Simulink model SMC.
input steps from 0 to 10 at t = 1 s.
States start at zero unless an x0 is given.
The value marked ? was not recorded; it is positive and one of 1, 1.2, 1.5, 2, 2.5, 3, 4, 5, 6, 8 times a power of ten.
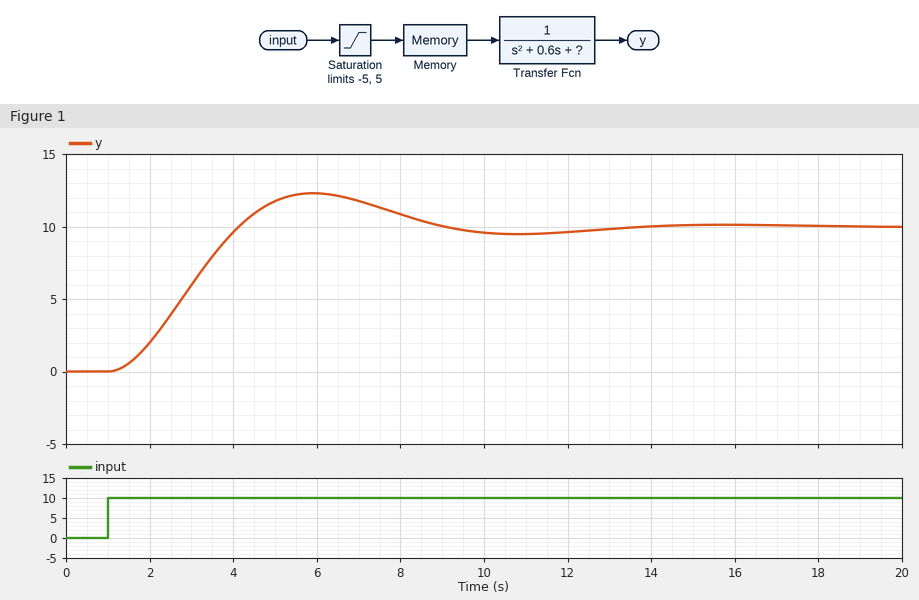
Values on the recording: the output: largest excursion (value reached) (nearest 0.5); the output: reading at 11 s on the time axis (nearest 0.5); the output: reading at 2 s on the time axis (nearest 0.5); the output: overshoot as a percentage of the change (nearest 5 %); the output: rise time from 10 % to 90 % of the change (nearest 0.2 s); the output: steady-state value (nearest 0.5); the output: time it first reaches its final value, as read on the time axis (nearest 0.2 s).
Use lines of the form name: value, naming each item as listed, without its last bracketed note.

the output: largest excursion (value reached): 12.5
the output: reading at 11 s on the time axis: 9.5
the output: reading at 2 s on the time axis: 2.0
the output: overshoot as a percentage of the change: 25 %
the output: rise time from 10 % to 90 % of the change: 2.2 s
the output: steady-state value: 10.0
the output: time it first reaches its final value, as read on the time axis: 4.2 s
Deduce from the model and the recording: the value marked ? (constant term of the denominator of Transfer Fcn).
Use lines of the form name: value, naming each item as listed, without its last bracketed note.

the value marked ?: 0.5
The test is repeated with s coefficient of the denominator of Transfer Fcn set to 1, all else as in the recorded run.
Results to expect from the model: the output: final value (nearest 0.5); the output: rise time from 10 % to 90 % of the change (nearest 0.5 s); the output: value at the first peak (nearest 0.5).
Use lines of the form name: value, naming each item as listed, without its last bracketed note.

the output: final value: 10.0
the output: rise time from 10 % to 90 % of the change: 3.0 s
the output: value at the first peak: 10.5
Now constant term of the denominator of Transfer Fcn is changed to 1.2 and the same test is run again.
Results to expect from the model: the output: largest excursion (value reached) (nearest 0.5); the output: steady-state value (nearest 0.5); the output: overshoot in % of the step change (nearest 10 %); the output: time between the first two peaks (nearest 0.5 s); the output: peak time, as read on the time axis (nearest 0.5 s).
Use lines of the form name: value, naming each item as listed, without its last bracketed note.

the output: largest excursion (value reached): 6.0
the output: steady-state value: 4.0
the output: overshoot in % of the step change: 40 %
the output: time between the first two peaks: 6.0 s
the output: peak time, as read on the time axis: 4.0 s
